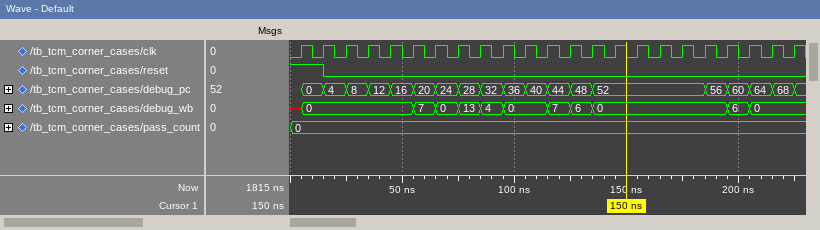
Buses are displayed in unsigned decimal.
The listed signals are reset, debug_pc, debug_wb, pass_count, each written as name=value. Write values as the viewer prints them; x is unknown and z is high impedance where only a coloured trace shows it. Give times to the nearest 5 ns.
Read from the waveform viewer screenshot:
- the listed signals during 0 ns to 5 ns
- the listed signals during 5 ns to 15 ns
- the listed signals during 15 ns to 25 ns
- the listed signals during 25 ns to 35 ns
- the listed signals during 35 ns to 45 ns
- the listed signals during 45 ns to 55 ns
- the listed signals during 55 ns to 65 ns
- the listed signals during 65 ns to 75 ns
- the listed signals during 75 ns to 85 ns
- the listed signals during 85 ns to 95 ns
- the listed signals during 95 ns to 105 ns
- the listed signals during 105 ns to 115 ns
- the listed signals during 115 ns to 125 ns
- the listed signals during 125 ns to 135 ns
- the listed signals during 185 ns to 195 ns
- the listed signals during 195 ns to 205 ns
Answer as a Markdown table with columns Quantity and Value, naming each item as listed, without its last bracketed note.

| Quantity | Value |
|---|---|
| the listed signals during 0 ns to 5 ns | reset=1, debug_pc=x, debug_wb=x, pass_count=0 |
| the listed signals during 5 ns to 15 ns | reset=1, debug_pc=0, debug_wb=0, pass_count=0 |
| the listed signals during 15 ns to 25 ns | reset=0, debug_pc=4, debug_wb=0, pass_count=0 |
| the listed signals during 25 ns to 35 ns | reset=0, debug_pc=8, debug_wb=0, pass_count=0 |
| the listed signals during 35 ns to 45 ns | reset=0, debug_pc=12, debug_wb=0, pass_count=0 |
| the listed signals during 45 ns to 55 ns | reset=0, debug_pc=16, debug_wb=0, pass_count=0 |
| the listed signals during 55 ns to 65 ns | reset=0, debug_pc=20, debug_wb=7, pass_count=0 |
| the listed signals during 65 ns to 75 ns | reset=0, debug_pc=24, debug_wb=0, pass_count=0 |
| the listed signals during 75 ns to 85 ns | reset=0, debug_pc=28, debug_wb=13, pass_count=0 |
| the listed signals during 85 ns to 95 ns | reset=0, debug_pc=32, debug_wb=4, pass_count=0 |
| the listed signals during 95 ns to 105 ns | reset=0, debug_pc=36, debug_wb=0, pass_count=0 |
| the listed signals during 105 ns to 115 ns | reset=0, debug_pc=40, debug_wb=0, pass_count=0 |
| the listed signals during 115 ns to 125 ns | reset=0, debug_pc=44, debug_wb=7, pass_count=0 |
| the listed signals during 125 ns to 135 ns | reset=0, debug_pc=48, debug_wb=6, pass_count=0 |
| the listed signals during 185 ns to 195 ns | reset=0, debug_pc=56, debug_wb=0, pass_count=0 |
| the listed signals during 195 ns to 205 ns | reset=0, debug_pc=60, debug_wb=6, pass_count=0 |
